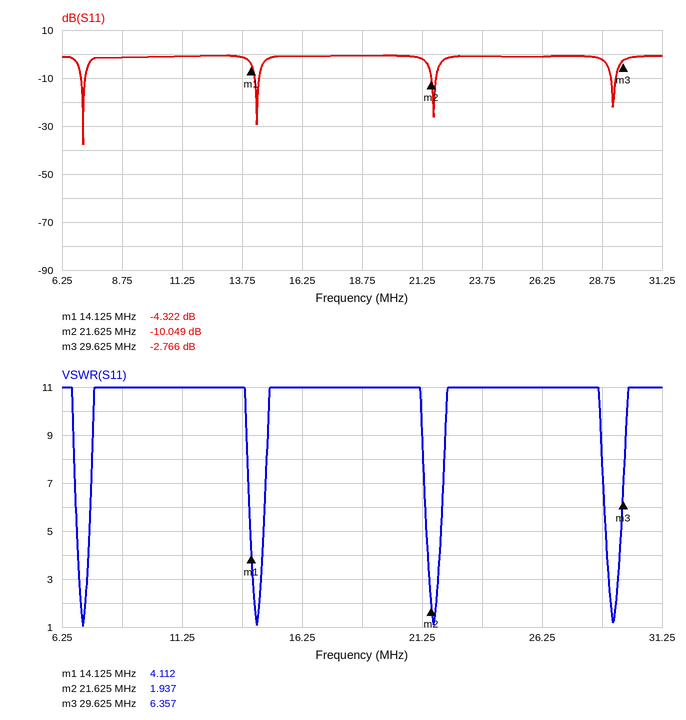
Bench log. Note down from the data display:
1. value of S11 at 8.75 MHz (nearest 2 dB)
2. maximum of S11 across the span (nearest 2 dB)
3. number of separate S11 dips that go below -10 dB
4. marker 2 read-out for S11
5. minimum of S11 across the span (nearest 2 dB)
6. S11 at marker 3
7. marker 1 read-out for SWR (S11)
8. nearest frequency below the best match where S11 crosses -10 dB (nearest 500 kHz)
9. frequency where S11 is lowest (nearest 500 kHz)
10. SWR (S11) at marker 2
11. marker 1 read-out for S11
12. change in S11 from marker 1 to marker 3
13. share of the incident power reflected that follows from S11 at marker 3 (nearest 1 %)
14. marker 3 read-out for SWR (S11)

-2 dB
0 dB
4
-10.049 dB
-38 dB
-2.766 dB
4.112
7.0 MHz
7.0 MHz
1.937
-4.322 dB
1.556 dB
53 %
6.357
